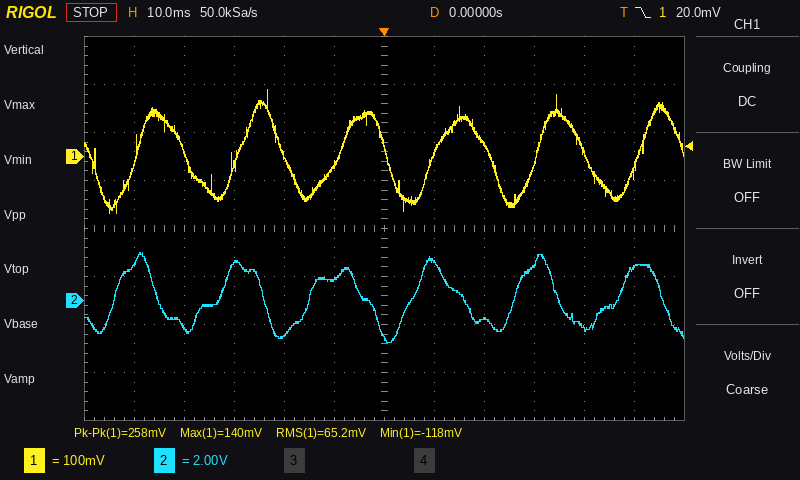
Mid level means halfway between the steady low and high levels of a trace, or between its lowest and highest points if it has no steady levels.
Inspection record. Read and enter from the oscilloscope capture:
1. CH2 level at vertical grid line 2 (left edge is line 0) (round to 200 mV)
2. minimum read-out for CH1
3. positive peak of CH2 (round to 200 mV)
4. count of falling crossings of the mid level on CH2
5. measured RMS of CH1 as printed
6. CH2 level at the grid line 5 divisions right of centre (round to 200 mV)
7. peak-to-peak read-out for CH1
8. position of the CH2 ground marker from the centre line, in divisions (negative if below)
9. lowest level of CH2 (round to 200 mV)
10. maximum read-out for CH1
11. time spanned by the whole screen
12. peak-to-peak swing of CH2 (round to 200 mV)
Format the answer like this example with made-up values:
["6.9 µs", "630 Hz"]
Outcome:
["-1.2 V", "-118 mV", "2.0 V", "6", "65.2 mV", "1.4 V", "258 mV", "-1.5 div", "-1.8 V", "140 mV", "120 ms", "3.8 V"]
